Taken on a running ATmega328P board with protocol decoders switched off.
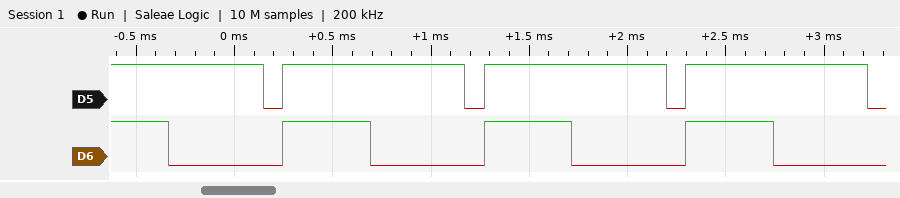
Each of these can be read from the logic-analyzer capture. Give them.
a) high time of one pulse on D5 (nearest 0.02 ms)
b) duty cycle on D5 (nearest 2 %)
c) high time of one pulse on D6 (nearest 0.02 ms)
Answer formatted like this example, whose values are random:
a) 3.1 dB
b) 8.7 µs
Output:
a) 0.92 ms
b) 90 %
c) 0.44 ms
